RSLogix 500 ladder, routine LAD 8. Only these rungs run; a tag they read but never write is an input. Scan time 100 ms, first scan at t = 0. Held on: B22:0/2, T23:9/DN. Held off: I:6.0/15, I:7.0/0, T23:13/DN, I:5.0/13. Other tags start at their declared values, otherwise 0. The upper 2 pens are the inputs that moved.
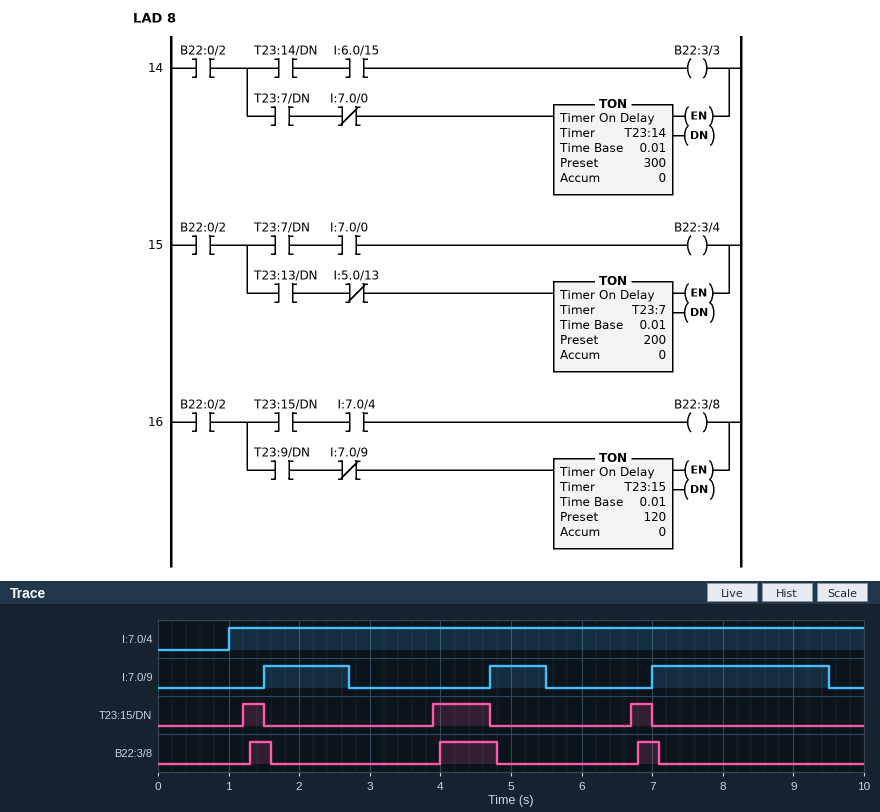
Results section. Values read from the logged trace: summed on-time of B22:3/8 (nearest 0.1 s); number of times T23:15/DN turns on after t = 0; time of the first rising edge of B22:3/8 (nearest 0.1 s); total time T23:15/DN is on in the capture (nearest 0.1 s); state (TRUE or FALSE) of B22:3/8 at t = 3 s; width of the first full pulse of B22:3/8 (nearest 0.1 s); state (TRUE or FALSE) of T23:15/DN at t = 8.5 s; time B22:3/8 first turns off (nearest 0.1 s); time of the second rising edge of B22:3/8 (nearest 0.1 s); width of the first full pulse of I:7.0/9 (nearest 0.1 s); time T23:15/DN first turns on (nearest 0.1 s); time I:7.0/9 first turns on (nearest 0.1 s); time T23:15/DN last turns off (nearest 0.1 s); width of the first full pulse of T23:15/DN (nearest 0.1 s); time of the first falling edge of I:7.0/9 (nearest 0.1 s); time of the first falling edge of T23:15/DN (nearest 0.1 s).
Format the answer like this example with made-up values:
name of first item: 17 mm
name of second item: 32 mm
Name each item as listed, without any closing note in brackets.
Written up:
summed on-time of B22:3/8: 1.4 s
number of times T23:15/DN turns on after t = 0: 3
time of the first rising edge of B22:3/8: 1.3 s
total time T23:15/DN is on in the capture: 1.4 s
state (TRUE or FALSE) of B22:3/8 at t = 3 s: FALSE
width of the first full pulse of B22:3/8: 0.3 s
state (TRUE or FALSE) of T23:15/DN at t = 8.5 s: FALSE
time B22:3/8 first turns off: 1.6 s
time of the second rising edge of B22:3/8: 4.0 s
width of the first full pulse of I:7.0/9: 1.2 s
time T23:15/DN first turns on: 1.2 s
time I:7.0/9 first turns on: 1.5 s
time T23:15/DN last turns off: 7.0 s
width of the first full pulse of T23:15/DN: 0.3 s
time of the first falling edge of I:7.0/9: 2.7 s
time of the first falling edge of T23:15/DN: 1.5 s
